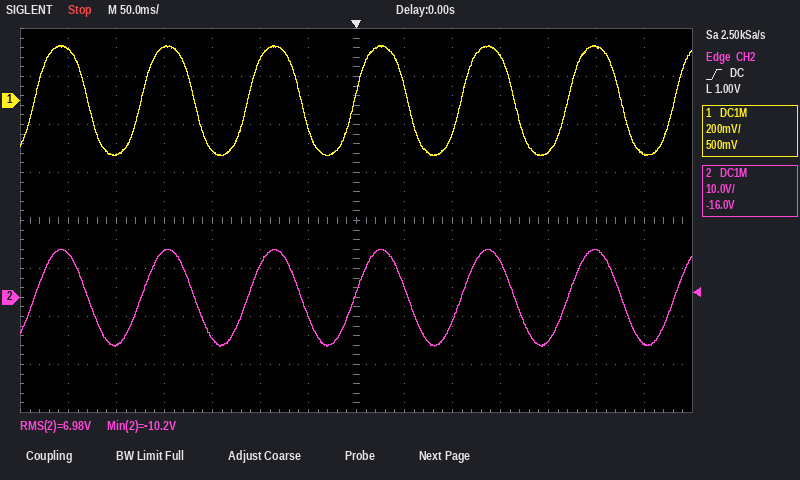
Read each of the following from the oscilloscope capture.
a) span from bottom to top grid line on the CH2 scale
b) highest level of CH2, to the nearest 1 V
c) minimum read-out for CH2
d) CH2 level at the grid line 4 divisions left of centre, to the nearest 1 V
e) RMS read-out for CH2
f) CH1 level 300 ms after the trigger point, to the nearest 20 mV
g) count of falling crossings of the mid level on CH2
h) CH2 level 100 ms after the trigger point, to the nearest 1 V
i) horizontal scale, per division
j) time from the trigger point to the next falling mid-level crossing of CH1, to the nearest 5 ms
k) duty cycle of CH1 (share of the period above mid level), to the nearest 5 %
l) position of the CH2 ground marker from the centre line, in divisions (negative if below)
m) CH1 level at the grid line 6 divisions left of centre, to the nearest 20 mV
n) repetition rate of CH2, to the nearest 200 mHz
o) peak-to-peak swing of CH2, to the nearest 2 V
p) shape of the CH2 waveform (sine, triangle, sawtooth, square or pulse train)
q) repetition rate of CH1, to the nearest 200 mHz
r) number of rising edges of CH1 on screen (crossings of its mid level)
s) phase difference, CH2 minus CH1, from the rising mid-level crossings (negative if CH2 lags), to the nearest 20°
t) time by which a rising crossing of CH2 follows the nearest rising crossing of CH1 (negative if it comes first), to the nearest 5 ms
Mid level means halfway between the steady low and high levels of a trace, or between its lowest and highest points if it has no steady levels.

80 V
10 V
-10.2 V
10 V
6.98 V
-220 mV
6
-5 V
50 ms
55 ms
50 %
-1.6 div
220 mV
9.0 Hz
20 V
sine
9.0 Hz
7
0°
0 ms
